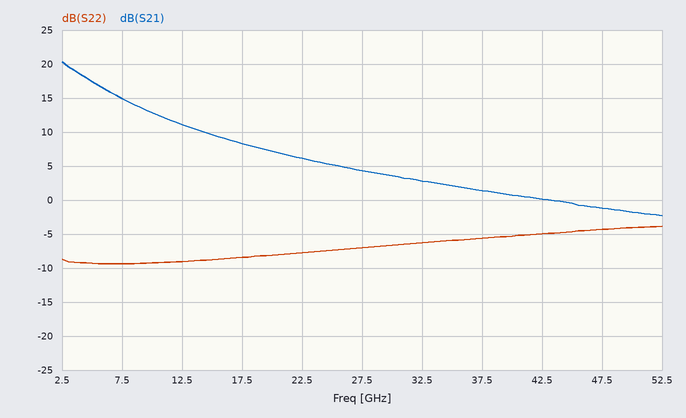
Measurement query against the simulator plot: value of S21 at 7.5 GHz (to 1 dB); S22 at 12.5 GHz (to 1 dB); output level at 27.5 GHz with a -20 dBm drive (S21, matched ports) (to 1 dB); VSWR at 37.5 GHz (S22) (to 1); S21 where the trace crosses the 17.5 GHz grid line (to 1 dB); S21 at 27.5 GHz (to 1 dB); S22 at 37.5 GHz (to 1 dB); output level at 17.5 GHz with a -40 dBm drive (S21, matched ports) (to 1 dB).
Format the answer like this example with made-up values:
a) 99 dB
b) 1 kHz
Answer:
a) 15 dB
b) -9 dB
c) -16 dBm
d) 3
e) 8 dB
f) 4 dB
g) -6 dB
h) -32 dBm
